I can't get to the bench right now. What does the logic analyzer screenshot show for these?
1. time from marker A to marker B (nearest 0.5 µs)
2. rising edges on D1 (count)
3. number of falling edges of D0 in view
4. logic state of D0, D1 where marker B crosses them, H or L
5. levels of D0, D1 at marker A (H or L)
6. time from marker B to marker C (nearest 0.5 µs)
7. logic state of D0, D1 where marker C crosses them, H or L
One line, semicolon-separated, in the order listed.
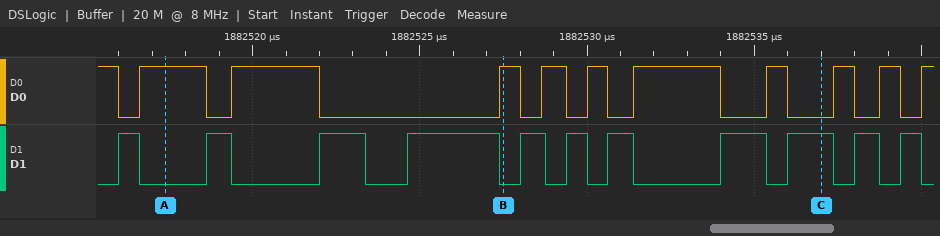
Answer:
10 µs; 11; 10; D0=H, D1=L; D0=H, D1=L; 9.5 µs; D0=L, D1=H
